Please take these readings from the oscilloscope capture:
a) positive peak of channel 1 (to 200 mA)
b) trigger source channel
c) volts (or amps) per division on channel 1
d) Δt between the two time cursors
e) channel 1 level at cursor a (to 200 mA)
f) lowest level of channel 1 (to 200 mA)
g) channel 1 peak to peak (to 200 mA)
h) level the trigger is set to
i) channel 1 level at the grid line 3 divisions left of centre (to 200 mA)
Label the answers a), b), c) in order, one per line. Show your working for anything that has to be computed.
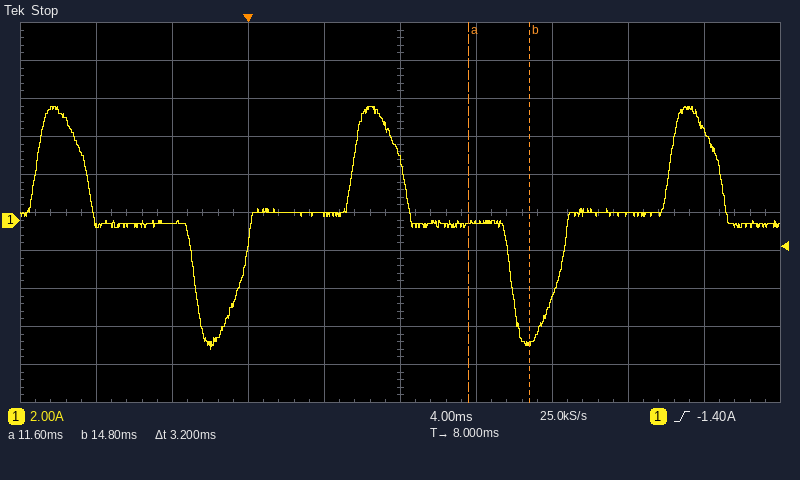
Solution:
a) 6.0 A
b) channel 1
c) 2 A
d) 3.2 ms
e) -200 mA
f) -6.8 A
g) 6.0 A − (-6.8 A) = 12.8 A
h) -1.40 A
i) -200 mA
